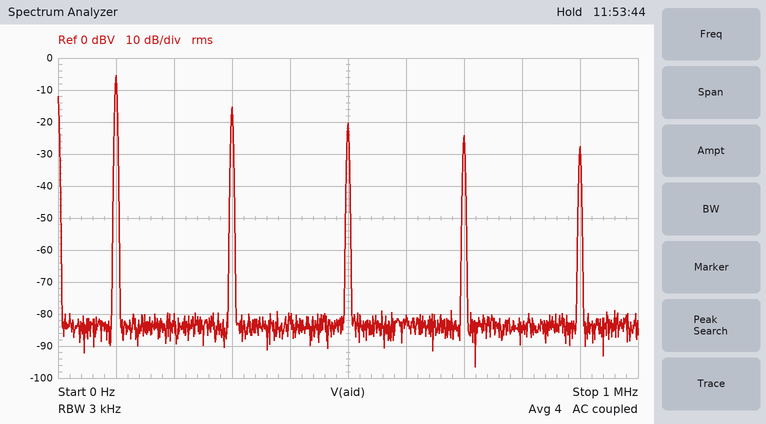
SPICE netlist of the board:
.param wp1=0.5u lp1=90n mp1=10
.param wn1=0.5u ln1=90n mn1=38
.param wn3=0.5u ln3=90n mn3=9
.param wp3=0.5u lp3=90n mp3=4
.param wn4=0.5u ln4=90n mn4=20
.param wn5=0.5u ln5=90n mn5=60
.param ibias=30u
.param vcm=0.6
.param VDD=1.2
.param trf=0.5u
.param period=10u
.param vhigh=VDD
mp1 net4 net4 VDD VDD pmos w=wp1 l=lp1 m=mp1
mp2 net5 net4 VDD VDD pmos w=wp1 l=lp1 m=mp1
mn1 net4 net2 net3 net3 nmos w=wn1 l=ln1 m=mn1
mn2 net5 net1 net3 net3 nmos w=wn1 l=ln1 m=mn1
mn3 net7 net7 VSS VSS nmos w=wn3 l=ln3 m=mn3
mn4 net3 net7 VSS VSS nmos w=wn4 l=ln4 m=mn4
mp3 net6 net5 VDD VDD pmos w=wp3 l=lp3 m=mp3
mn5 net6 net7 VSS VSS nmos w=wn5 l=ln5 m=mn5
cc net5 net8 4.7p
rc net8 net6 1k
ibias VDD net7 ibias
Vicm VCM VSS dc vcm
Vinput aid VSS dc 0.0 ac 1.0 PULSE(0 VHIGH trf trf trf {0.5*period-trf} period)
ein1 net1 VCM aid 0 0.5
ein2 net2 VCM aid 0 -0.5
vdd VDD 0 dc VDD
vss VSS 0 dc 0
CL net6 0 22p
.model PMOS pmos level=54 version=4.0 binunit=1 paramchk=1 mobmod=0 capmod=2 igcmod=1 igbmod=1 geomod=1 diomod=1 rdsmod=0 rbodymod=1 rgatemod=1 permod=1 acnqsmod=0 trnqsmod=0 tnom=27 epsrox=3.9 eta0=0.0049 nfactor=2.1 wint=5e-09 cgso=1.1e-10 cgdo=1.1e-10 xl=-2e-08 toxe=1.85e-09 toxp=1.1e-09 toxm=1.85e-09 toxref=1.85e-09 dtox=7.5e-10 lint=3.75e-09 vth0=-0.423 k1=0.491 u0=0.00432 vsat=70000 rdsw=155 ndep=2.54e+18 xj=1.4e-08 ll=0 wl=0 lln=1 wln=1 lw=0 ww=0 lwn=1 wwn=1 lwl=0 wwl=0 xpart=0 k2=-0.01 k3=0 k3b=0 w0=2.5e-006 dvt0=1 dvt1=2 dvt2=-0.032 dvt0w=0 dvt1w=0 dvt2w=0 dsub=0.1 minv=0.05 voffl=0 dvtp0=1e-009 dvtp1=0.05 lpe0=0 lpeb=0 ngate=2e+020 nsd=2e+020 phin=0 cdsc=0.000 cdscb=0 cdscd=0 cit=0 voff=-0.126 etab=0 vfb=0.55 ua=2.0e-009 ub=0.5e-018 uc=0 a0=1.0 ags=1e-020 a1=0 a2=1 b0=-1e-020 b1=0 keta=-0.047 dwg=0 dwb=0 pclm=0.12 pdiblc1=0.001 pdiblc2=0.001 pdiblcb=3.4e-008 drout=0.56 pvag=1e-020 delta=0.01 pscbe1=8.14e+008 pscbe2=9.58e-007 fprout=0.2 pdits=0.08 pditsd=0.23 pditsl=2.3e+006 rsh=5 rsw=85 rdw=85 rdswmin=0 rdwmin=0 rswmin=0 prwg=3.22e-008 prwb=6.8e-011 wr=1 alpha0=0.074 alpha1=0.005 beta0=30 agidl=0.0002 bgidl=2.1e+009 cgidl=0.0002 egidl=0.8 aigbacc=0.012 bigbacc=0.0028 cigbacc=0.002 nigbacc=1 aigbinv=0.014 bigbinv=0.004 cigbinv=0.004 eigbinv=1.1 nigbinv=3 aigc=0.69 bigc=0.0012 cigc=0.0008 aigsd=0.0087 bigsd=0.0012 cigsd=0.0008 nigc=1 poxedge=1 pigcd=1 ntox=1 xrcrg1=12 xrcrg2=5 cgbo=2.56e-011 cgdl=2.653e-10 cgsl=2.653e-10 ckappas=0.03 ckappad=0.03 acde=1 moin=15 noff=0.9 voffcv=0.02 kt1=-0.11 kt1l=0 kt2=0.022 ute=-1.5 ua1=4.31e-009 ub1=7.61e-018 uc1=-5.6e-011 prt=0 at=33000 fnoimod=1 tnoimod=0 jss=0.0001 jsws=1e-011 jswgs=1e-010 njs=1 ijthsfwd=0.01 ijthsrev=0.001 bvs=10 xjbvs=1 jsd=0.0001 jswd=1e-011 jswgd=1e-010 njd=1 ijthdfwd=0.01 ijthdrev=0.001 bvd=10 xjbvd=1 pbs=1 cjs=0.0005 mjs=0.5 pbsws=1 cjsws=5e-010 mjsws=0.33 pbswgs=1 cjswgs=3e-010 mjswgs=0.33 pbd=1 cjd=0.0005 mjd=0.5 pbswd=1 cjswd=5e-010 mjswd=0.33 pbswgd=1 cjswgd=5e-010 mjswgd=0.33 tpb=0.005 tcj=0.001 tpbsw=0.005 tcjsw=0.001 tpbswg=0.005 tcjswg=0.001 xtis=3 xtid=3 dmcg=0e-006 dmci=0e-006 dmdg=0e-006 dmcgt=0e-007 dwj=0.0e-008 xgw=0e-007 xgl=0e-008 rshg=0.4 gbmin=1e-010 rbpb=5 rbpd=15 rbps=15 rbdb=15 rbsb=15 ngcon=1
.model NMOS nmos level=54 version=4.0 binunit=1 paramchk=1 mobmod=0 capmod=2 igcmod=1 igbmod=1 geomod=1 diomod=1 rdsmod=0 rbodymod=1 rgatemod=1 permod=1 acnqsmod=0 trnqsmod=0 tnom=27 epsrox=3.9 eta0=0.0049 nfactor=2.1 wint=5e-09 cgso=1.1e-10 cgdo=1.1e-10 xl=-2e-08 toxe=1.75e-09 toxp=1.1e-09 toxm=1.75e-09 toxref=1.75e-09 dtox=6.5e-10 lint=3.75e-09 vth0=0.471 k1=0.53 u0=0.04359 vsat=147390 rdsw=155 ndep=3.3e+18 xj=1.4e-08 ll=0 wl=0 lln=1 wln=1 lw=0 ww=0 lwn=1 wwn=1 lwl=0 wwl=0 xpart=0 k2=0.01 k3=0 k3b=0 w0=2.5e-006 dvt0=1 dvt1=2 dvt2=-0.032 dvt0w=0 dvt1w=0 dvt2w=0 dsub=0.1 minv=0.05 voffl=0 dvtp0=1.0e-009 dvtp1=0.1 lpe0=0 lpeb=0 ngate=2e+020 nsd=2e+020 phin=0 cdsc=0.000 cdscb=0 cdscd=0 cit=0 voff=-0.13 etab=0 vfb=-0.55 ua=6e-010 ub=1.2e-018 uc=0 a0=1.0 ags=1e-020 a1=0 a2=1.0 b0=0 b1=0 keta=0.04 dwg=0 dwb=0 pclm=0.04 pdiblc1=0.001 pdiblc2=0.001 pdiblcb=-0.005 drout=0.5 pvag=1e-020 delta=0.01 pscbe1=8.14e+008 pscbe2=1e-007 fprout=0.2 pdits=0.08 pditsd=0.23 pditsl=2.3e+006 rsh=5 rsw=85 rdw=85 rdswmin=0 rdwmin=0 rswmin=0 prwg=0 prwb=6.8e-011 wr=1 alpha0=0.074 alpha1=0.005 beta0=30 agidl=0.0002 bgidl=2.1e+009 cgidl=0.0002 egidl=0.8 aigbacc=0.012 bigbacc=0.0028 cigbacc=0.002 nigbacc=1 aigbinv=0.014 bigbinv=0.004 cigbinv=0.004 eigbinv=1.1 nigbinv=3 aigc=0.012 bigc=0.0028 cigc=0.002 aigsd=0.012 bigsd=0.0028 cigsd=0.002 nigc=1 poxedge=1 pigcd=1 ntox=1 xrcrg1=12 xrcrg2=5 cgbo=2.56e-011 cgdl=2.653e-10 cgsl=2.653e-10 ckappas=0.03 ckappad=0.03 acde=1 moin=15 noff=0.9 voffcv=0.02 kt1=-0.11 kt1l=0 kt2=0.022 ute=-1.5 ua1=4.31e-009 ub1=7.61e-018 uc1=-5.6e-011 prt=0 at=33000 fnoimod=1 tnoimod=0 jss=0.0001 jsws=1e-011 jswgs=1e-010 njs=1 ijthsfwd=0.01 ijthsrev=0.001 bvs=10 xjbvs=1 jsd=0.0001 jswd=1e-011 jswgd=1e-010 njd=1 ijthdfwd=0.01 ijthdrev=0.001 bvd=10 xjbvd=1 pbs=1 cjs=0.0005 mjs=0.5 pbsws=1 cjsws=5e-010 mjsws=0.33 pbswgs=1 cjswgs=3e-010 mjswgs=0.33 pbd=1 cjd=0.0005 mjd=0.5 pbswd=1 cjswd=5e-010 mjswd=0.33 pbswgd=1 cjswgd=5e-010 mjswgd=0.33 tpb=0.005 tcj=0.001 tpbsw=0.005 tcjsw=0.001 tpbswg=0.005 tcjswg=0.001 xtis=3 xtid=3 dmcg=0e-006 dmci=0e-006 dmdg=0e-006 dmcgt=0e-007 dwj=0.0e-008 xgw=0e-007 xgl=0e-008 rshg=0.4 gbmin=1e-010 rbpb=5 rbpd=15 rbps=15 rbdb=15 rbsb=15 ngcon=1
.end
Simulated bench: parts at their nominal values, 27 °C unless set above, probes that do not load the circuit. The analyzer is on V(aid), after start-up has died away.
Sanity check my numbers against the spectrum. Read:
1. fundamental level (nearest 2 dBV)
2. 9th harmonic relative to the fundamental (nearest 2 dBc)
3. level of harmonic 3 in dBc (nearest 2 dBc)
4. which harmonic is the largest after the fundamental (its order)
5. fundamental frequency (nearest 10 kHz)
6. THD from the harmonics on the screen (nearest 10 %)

-6 dBV
-22 dBc
-10 dBc
3
100 kHz
40 %
